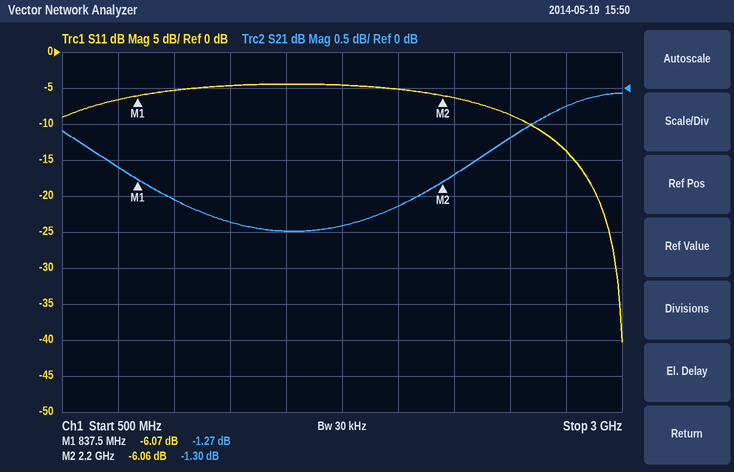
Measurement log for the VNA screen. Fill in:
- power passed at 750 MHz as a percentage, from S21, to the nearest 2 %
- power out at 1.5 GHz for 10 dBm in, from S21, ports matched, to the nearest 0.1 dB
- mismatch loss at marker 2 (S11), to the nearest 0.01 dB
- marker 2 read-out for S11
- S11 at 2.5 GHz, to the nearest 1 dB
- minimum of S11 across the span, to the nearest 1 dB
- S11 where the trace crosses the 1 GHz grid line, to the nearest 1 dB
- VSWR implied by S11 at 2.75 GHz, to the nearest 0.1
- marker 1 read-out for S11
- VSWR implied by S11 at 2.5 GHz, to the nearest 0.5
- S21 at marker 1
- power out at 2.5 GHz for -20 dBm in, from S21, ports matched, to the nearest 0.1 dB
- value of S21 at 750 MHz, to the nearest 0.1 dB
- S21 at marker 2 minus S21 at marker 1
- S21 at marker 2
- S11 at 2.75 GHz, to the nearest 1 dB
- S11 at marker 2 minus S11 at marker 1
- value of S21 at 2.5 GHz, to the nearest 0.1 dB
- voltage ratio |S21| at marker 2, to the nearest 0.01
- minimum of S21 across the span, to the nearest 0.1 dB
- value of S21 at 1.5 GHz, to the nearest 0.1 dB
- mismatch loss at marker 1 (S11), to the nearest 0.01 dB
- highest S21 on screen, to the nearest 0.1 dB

78 %
8.0 dBm
1.24 dB
-6.06 dB
-9 dB
-40 dB
-5 dB
1.5
-6.07 dB
2.0
-1.27 dB
-20.7 dBm
-1.1 dB
-0.03 dB
-1.30 dB
-14 dB
0.01 dB
-0.7 dB
0.86
-2.0 dB
-2.0 dB
1.23 dB
-0.1 dB
